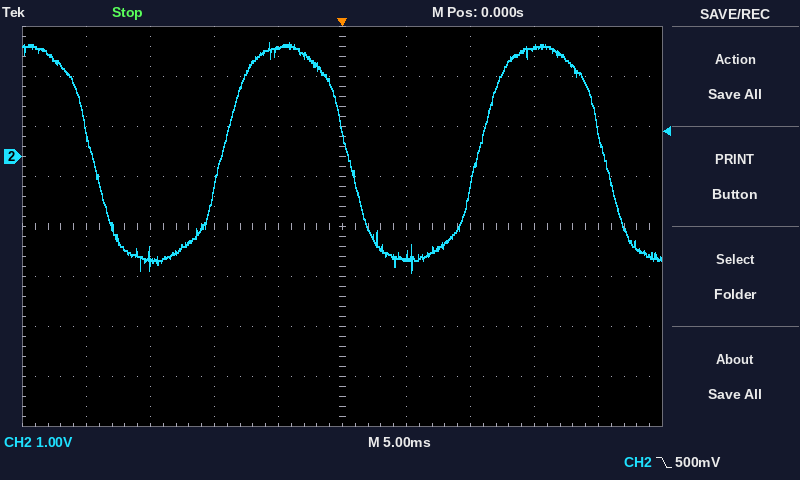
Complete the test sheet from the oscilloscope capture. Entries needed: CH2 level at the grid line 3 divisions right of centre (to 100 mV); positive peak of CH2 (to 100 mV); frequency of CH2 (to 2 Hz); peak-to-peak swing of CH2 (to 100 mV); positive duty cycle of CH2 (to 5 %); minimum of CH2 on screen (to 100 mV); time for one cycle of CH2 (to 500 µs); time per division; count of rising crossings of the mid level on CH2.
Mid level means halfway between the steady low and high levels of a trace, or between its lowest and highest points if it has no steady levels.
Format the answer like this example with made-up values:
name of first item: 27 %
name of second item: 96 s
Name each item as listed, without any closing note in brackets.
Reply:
CH2 level at the grid line 3 divisions right of centre: 2.2 V
positive peak of CH2: 2.3 V
frequency of CH2: 50 Hz
peak-to-peak swing of CH2: 4.6 V
positive duty cycle of CH2: 50 %
minimum of CH2 on screen: -2.3 V
time for one cycle of CH2: 20.0 ms
time per division: 5 ms
count of rising crossings of the mid level on CH2: 2
